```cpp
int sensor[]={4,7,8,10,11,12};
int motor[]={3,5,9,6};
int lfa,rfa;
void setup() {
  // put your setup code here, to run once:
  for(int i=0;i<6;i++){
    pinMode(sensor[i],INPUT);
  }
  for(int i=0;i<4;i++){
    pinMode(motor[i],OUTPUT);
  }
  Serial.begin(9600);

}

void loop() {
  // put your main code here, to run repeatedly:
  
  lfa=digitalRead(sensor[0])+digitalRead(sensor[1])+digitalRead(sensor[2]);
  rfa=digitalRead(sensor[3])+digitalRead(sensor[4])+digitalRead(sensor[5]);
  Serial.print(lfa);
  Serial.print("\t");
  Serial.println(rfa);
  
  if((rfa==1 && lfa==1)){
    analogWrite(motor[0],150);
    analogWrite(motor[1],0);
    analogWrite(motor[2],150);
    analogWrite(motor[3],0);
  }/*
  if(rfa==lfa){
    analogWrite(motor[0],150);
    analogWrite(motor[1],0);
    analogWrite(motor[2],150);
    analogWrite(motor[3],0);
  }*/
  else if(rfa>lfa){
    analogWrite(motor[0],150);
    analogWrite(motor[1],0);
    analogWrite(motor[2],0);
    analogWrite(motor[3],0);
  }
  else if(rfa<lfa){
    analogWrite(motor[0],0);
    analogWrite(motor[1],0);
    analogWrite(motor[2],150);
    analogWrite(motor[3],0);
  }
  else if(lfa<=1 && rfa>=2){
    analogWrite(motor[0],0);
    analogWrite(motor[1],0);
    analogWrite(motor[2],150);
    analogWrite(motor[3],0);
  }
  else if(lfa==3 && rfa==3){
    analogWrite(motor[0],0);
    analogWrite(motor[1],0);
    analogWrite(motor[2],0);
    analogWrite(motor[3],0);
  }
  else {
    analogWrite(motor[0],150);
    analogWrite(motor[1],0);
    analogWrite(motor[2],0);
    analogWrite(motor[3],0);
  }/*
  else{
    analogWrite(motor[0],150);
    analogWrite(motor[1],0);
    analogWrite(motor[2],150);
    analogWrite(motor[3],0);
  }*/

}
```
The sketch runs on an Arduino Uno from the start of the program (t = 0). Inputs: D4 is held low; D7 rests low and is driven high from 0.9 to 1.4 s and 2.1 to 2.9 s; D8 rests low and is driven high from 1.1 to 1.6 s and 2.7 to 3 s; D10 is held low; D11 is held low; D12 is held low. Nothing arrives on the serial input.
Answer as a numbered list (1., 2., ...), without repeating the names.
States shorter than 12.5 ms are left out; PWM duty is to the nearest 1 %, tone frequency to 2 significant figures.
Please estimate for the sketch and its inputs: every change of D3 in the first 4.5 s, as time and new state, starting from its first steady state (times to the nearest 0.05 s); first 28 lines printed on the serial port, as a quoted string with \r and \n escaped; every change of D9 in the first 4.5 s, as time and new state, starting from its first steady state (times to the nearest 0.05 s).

1. 0 s PWM 59 %; 0.9 s low; 1.6 s PWM 59 %; 2.1 s low; 3 s PWM 59 %
2. "0\t0\r\n0\t0\r\n0\t0\r\n0\t0\r\n0\t0\r\n0\t0\r\n0\t0\r\n0\t0\r\n0\t0\r\n0\t0\r\n0\t0\r\n0\t0\r\n0\t0\r\n0\t0\r\n0\t0\r\n0\t0\r\n0\t0\r\n0\t0\r\n0\t0\r\n0\t0\r\n0\t0\r\n0\t0\r\n0\t0\r\n0\t0\r\n0\t0\r\n0\t0\r\n0\t0\r\n0\t0\r\n"
3. 0 s low; 0.9 s PWM 59 %; 1.6 s low; 2.1 s PWM 59 %; 3 s low
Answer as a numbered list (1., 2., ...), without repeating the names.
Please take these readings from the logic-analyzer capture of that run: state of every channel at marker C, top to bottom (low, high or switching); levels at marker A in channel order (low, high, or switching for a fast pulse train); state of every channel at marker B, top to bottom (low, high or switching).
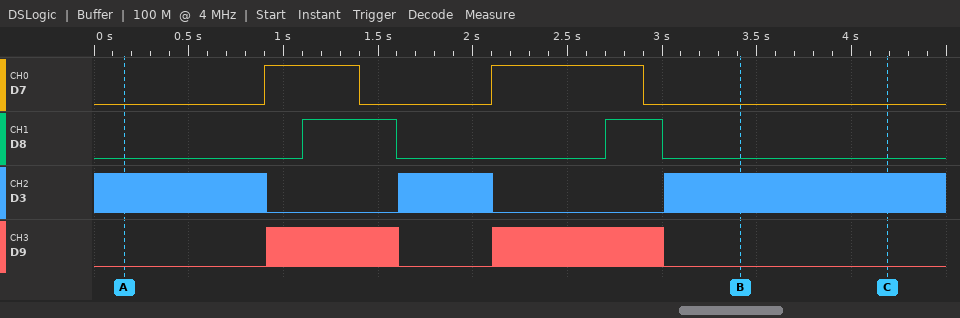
1. D7 low, D8 low, D3 switching, D9 low
2. D7 low, D8 low, D3 switching, D9 low
3. D7 low, D8 low, D3 switching, D9 low
